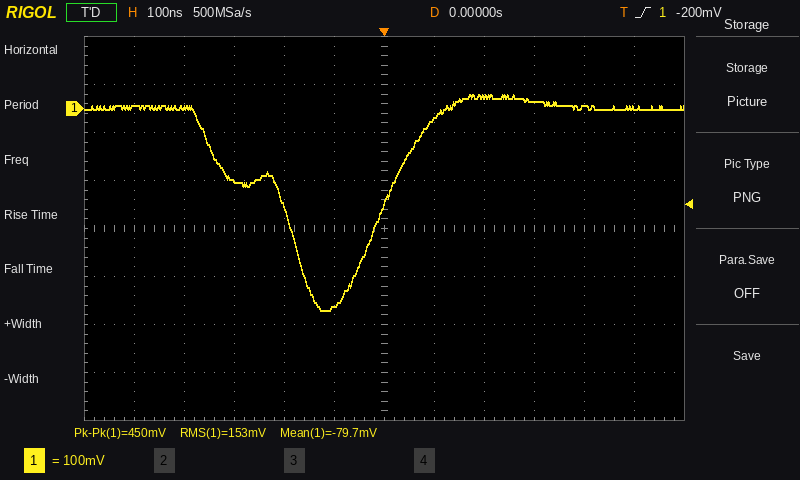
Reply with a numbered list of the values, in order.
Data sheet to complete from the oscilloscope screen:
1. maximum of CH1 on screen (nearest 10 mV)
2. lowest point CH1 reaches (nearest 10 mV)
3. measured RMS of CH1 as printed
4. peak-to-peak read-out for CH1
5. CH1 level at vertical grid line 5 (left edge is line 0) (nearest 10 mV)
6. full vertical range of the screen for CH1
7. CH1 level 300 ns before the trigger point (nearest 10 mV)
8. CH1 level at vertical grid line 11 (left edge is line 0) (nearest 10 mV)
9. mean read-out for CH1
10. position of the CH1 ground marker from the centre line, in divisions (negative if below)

1. 30 mV
2. -420 mV
3. 153 mV
4. 450 mV
5. -410 mV
6. 800 mV
7. -150 mV
8. 0 mV
9. -79.7 mV
10. +2.5 div
